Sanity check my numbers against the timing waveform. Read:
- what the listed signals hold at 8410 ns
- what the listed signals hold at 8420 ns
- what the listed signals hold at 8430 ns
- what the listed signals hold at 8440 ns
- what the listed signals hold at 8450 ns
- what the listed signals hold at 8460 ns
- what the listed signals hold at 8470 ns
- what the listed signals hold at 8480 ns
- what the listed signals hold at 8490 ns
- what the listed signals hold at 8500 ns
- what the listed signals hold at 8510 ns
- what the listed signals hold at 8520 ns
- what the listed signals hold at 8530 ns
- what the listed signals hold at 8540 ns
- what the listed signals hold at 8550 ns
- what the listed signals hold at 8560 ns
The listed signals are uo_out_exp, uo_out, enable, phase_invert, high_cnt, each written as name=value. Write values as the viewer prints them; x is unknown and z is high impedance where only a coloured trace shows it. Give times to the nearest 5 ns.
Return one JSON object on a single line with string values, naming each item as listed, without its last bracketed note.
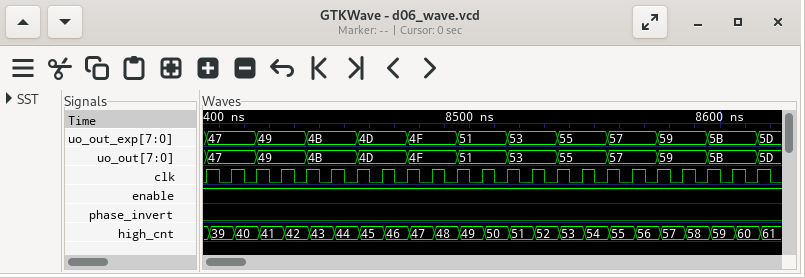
{"what the listed signals hold at 8410 ns": "uo_out_exp=47, uo_out=47, enable=1, phase_invert=0, high_cnt=40", "what the listed signals hold at 8420 ns": "uo_out_exp=49, uo_out=49, enable=1, phase_invert=0, high_cnt=41", "what the listed signals hold at 8430 ns": "uo_out_exp=49, uo_out=49, enable=1, phase_invert=0, high_cnt=42", "what the listed signals hold at 8440 ns": "uo_out_exp=4B, uo_out=4B, enable=1, phase_invert=0, high_cnt=43", "what the listed signals hold at 8450 ns": "uo_out_exp=4B, uo_out=4B, enable=1, phase_invert=0, high_cnt=44", "what the listed signals hold at 8460 ns": "uo_out_exp=4D, uo_out=4D, enable=1, phase_invert=0, high_cnt=45", "what the listed signals hold at 8470 ns": "uo_out_exp=4D, uo_out=4D, enable=1, phase_invert=0, high_cnt=46", "what the listed signals hold at 8480 ns": "uo_out_exp=4F, uo_out=4F, enable=1, phase_invert=0, high_cnt=47", "what the listed signals hold at 8490 ns": "uo_out_exp=4F, uo_out=4F, enable=1, phase_invert=0, high_cnt=48", "what the listed signals hold at 8500 ns": "uo_out_exp=51, uo_out=51, enable=1, phase_invert=0, high_cnt=49", "what the listed signals hold at 8510 ns": "uo_out_exp=51, uo_out=51, enable=1, phase_invert=0, high_cnt=50", "what the listed signals hold at 8520 ns": "uo_out_exp=53, uo_out=53, enable=1, phase_invert=0, high_cnt=51", "what the listed signals hold at 8530 ns": "uo_out_exp=53, uo_out=53, enable=1, phase_invert=0, high_cnt=52", "what the listed signals hold at 8540 ns": "uo_out_exp=55, uo_out=55, enable=1, phase_invert=0, high_cnt=53", "what the listed signals hold at 8550 ns": "uo_out_exp=55, uo_out=55, enable=1, phase_invert=0, high_cnt=54", "what the listed signals hold at 8560 ns": "uo_out_exp=57, uo_out=57, enable=1, phase_invert=0, high_cnt=55"}
